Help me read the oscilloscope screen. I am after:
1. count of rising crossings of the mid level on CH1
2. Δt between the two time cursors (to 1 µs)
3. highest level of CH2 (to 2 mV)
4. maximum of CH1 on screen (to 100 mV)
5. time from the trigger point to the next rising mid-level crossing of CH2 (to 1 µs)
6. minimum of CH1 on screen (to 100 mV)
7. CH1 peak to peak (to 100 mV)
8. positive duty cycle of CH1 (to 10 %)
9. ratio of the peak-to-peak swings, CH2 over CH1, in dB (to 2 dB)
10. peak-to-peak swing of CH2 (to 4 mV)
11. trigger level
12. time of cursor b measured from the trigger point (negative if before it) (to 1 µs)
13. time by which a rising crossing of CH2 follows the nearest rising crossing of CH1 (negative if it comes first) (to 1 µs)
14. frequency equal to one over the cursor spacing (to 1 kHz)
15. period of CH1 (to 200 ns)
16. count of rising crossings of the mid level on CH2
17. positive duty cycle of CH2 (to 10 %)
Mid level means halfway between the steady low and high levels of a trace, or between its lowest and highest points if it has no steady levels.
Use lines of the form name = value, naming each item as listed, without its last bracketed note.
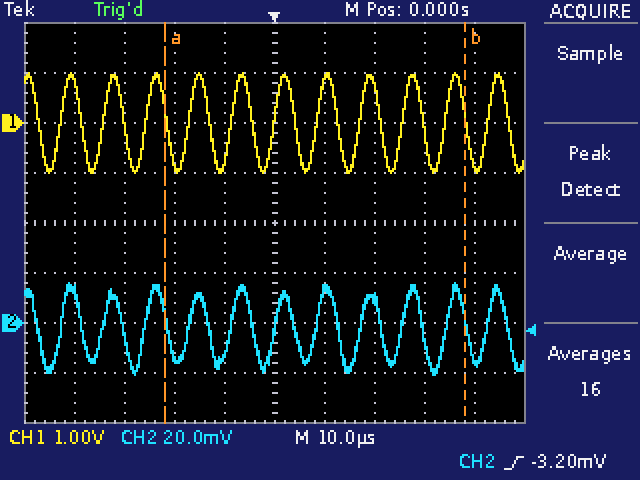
count of rising crossings of the mid level on CH1 = 11
Δt between the two time cursors = 60 µs
highest level of CH2 = 16 mV
maximum of CH1 on screen = 1.0 V
time from the trigger point to the next rising mid-level crossing of CH2 = 8 µs
minimum of CH1 on screen = -1.0 V
CH1 peak to peak = 2.0 V
positive duty cycle of CH1 = 50 %
ratio of the peak-to-peak swings, CH2 over CH1, in dB = -34 dB
peak-to-peak swing of CH2 = 36 mV
trigger level = -3.20 mV
time of cursor b measured from the trigger point (negative if before it) = +38 µs
time by which a rising crossing of CH2 follows the nearest rising crossing of CH1 (negative if it comes first) = 0 µs
frequency equal to one over the cursor spacing = 17 kHz
period of CH1 = 8.6 µs
count of rising crossings of the mid level on CH2 = 11
positive duty cycle of CH2 = 50 %
